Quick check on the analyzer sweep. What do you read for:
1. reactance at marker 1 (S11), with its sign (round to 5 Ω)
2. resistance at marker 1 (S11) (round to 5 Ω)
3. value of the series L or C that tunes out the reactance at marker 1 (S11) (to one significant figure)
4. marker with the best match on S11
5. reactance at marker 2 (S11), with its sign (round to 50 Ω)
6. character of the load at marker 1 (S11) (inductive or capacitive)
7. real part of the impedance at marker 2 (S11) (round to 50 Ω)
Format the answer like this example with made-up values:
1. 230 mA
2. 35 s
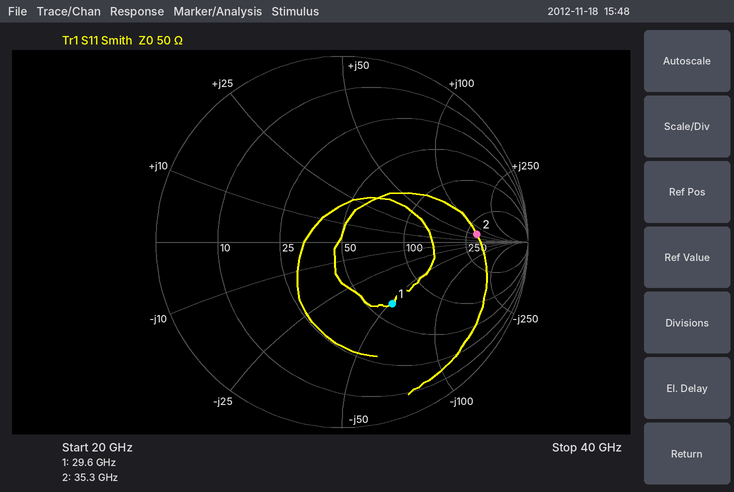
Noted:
1. -50 Ω
2. 65 Ω
3. 300 pH
4. marker 1
5. +50 Ω
6. capacitive
7. 300 Ω
